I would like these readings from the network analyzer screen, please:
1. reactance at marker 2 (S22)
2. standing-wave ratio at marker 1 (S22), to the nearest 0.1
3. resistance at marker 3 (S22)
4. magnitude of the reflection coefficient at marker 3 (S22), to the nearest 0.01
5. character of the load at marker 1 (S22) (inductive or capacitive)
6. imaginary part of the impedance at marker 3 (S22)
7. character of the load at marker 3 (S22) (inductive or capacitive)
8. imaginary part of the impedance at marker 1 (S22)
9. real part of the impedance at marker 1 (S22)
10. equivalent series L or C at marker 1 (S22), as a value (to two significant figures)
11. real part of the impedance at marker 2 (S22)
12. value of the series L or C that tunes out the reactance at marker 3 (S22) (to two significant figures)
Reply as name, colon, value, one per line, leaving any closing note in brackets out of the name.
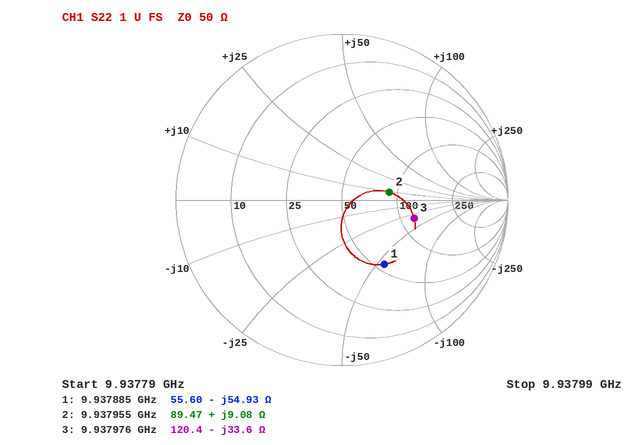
reactance at marker 2: +9.08 Ω
standing-wave ratio at marker 1 (S22), to the nearest 0.1: 2.7
resistance at marker 3: 120.4 Ω
magnitude of the reflection coefficient at marker 3 (S22), to the nearest 0.01: 0.45
character of the load at marker 1 (S22): capacitive
imaginary part of the impedance at marker 3: -33.6 Ω
character of the load at marker 3 (S22): capacitive
imaginary part of the impedance at marker 1: -54.93 Ω
real part of the impedance at marker 1: 55.60 Ω
equivalent series L or C at marker 1 (S22), as a value: 290 fF
real part of the impedance at marker 2: 89.47 Ω
value of the series L or C that tunes out the reactance at marker 3 (S22): 540 pH
